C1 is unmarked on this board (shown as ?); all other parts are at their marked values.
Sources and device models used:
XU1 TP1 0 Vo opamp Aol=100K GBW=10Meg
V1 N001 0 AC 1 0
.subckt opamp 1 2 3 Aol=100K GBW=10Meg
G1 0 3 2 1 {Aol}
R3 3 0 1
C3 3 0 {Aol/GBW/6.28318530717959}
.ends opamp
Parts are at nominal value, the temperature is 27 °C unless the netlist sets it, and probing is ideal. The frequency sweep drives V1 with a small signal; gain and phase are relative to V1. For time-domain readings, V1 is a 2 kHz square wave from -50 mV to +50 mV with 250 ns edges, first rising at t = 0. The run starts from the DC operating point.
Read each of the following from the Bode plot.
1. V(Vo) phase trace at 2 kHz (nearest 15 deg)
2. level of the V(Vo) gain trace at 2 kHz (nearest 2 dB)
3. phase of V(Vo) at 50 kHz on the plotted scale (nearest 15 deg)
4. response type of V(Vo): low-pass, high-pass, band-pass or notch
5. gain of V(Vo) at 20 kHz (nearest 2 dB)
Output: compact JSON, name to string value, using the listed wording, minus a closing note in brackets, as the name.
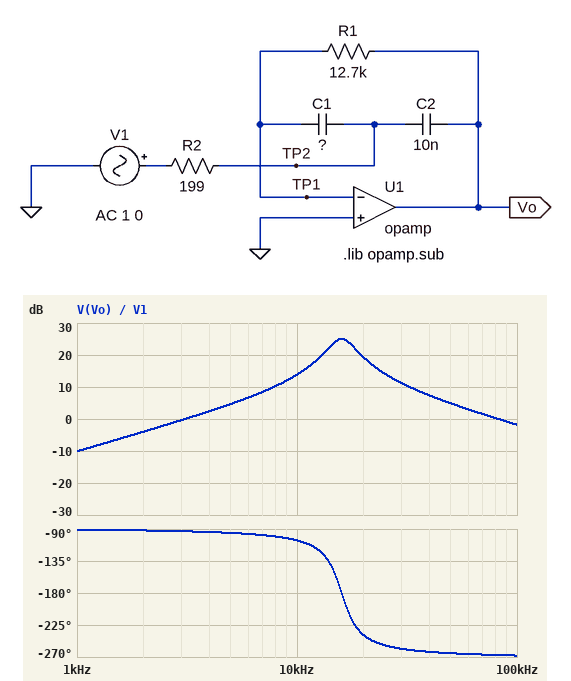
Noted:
{"V(Vo) phase trace at 2 kHz": "-90 deg", "level of the V(Vo) gain trace at 2 kHz": "-4 dB", "phase of V(Vo) at 50 kHz on the plotted scale": "-270 deg", "response type of V(Vo): low-pass, high-pass, band-pass or notch": "band-pass", "gain of V(Vo) at 20 kHz": "20 dB"}
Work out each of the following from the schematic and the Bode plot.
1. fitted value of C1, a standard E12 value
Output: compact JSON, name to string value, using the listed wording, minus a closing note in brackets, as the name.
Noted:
{"fitted value of C1, a standard E12 value": "3.9 nF"}
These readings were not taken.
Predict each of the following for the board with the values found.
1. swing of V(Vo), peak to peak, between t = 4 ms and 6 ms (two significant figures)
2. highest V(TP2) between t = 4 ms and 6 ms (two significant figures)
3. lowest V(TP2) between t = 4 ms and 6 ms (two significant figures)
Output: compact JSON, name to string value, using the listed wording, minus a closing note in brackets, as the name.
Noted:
{"swing of V(Vo), peak to peak, between t = 4 ms and 6 ms": "790 mV", "highest V(TP2) between t = 4 ms and 6 ms": "110 mV", "lowest V(TP2) between t = 4 ms and 6 ms": "-110 mV"}
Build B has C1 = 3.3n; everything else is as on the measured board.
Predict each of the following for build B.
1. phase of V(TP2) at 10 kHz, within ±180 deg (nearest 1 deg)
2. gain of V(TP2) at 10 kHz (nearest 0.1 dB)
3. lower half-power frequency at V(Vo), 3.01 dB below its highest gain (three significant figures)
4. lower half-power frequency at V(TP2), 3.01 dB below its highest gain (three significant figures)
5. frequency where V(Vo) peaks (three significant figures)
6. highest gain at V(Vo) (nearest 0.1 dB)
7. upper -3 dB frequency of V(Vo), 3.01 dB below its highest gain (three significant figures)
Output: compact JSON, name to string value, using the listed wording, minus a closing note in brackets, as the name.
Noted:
{"phase of V(TP2) at 10 kHz, within ±180 deg": "-14 deg", "gain of V(TP2) at 10 kHz": "3.2 dB", "lower half-power frequency at V(Vo), 3.01 dB below its highest gain": "15.0 kHz", "lower half-power frequency at V(TP2), 3.01 dB below its highest gain": "14.2 kHz", "frequency where V(Vo) peaks": "17.4 kHz", "highest gain at V(Vo)": "24.0 dB", "upper -3 dB frequency of V(Vo), 3.01 dB below its highest gain": "20.0 kHz"}
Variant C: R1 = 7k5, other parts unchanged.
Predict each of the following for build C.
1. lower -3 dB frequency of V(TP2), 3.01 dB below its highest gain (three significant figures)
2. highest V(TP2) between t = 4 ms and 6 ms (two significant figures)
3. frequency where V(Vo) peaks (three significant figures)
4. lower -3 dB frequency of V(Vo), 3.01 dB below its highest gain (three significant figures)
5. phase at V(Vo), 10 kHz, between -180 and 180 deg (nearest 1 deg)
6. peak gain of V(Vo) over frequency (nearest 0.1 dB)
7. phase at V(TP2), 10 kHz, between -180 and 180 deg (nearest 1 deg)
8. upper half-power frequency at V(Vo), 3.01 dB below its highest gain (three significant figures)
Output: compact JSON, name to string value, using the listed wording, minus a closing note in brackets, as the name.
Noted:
{"lower -3 dB frequency of V(TP2), 3.01 dB below its highest gain": "15.8 kHz", "highest V(TP2) between t = 4 ms and 6 ms": "110 mV", "frequency where V(Vo) peaks": "20.8 kHz", "lower -3 dB frequency of V(Vo), 3.01 dB below its highest gain": "17.4 kHz", "phase at V(Vo), 10 kHz, between -180 and 180 deg": "-103 deg", "peak gain of V(Vo) over frequency": "20.5 dB", "phase at V(TP2), 10 kHz, between -180 and 180 deg": "-13 deg", "upper half-power frequency at V(Vo), 3.01 dB below its highest gain": "24.9 kHz"}
